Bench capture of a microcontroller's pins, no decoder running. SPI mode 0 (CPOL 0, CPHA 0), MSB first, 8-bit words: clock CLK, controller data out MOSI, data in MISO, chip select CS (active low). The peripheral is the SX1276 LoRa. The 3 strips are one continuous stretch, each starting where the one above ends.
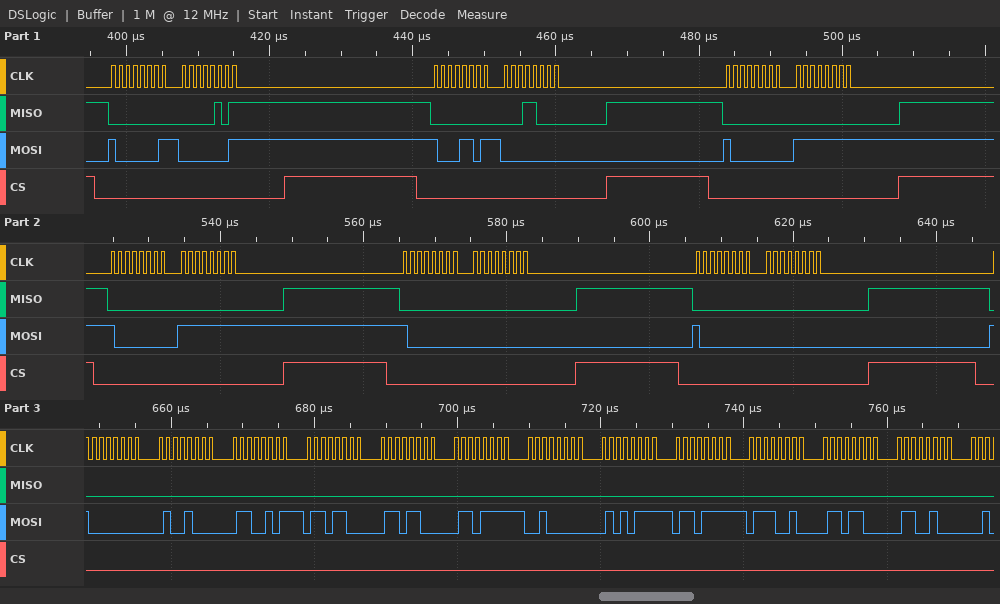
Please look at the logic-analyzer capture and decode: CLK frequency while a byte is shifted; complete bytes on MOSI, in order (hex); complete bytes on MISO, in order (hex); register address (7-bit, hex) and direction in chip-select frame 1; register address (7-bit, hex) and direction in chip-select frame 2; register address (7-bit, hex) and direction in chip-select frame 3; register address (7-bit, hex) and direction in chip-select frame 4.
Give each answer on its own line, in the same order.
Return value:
1 MHz
81 01 8D 00 80 FF 80 FF 80 00 80 00 80 48 65 6C 6C 6F 20 57 6F 72 6C 64
00 05 00 18 00 00 00 00 00 00 00 00 00 00 00 00 00 00 00 00 00 00 00 00
0x01 write
0x0D write
0x00 write
0x00 write
